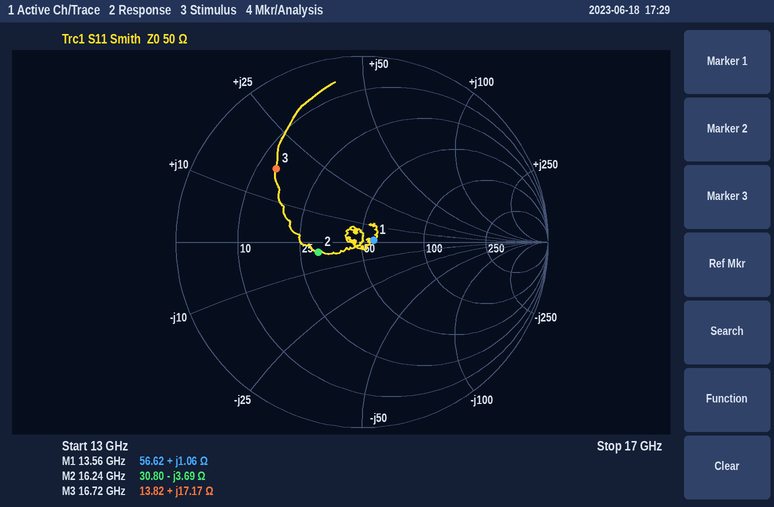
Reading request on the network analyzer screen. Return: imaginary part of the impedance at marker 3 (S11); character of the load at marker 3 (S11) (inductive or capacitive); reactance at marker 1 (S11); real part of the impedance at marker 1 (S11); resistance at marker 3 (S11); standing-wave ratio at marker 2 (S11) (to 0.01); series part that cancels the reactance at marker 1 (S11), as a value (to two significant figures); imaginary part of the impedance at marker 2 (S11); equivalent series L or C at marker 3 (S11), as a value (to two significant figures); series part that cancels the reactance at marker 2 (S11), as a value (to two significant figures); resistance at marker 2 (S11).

+17.17 Ω
inductive
+1.06 Ω
56.62 Ω
13.82 Ω
1.64
11 pF
-3.69 Ω
160 pH
36 pH
30.80 Ω
